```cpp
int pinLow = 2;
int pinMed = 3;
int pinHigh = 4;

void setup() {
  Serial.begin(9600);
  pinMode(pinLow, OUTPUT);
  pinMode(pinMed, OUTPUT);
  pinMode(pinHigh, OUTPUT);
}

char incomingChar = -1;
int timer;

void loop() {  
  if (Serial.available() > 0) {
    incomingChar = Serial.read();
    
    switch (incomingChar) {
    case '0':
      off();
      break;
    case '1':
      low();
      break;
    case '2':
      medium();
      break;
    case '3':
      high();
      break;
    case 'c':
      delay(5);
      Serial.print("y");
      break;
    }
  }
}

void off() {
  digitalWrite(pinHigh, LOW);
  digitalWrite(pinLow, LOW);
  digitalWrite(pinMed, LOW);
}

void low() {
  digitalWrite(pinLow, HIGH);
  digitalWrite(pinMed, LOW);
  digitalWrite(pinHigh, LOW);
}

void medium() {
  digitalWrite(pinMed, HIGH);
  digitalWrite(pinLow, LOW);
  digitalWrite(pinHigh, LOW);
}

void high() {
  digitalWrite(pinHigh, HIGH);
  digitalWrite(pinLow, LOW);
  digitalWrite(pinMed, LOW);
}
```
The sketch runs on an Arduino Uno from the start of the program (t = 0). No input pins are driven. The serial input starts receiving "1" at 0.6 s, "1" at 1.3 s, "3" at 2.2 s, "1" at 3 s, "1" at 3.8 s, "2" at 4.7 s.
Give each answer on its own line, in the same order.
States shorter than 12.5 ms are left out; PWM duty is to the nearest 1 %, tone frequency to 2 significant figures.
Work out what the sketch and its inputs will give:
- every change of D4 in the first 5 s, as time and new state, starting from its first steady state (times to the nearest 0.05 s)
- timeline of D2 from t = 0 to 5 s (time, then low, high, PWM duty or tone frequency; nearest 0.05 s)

0 s low; 2.2 s high; 3 s low
0 s low; 0.6 s high; 2.2 s low; 3 s high; 4.7 s low
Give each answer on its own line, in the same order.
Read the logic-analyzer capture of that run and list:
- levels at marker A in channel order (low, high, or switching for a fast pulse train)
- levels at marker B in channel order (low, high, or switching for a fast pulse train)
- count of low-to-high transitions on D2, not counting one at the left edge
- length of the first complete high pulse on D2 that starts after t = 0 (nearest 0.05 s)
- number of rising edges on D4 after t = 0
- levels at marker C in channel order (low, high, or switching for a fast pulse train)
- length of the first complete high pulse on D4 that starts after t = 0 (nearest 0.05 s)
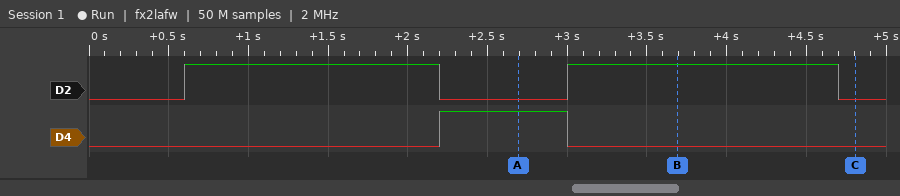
D2 low, D4 high
D2 high, D4 low
2
1.60 s
1
D2 low, D4 low
0.80 s
